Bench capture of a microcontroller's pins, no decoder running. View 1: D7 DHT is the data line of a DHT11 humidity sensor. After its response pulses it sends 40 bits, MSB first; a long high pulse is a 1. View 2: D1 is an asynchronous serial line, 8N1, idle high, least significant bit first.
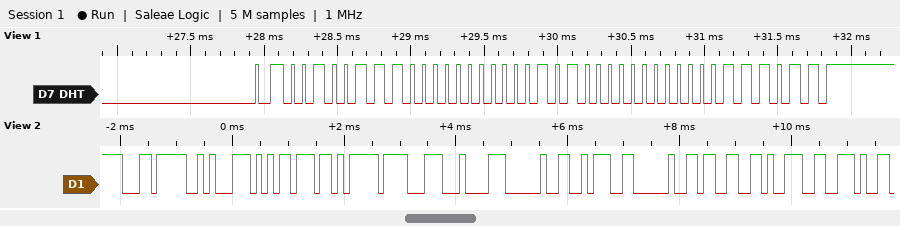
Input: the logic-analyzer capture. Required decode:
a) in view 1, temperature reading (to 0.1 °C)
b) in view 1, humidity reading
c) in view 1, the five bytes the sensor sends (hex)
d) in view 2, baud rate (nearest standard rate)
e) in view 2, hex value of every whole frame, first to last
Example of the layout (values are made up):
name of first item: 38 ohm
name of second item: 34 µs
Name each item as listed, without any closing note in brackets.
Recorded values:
in view 1, temperature reading: 20.0 °C
in view 1, humidity reading: 39 %
in view 1, the five bytes the sensor sends: 27 00 14 00 3B
in view 2, baud rate: 9600 baud
in view 2, hex value of every whole frame, first to last: EC 8A B5 EB 8F 84 20 3A 20 33 39 2E
